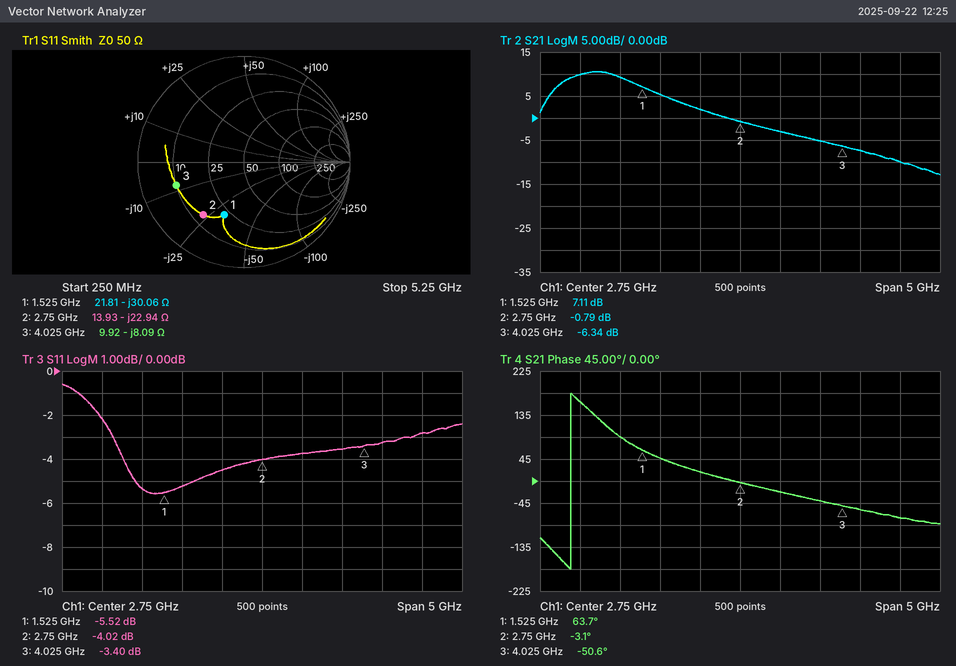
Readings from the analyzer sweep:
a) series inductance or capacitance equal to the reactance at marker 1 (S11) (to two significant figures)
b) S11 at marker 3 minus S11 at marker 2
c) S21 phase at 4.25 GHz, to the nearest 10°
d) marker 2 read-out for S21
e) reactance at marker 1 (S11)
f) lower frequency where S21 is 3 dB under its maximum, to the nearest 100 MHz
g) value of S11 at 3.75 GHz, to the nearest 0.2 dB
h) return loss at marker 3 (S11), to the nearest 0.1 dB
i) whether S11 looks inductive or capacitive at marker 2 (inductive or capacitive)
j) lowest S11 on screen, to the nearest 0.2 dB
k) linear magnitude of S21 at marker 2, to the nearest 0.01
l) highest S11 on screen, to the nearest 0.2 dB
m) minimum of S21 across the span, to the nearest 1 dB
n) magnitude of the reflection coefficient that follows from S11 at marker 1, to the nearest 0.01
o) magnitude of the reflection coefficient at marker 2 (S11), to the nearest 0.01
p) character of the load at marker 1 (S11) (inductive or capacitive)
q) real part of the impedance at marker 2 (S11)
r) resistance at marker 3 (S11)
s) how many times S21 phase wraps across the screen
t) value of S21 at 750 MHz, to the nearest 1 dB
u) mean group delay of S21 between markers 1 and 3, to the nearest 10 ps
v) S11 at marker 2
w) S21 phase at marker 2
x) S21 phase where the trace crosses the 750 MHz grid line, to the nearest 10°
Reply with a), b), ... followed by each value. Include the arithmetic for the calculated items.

a) C = 1/(2π × 1.525 GHz × 30.06 Ω) ≈ 3.5 pF
b) -3.4 − (-4.02) = 0.62 dB
c) -60°
d) -0.79 dB
e) -30.06 Ω
f) 500 MHz
g) -3.6 dB
h) 3.4 dB
i) capacitive
j) -5.6 dB
k) 10^(-0.79/20) ≈ 0.91
l) -0.6 dB
m) -13 dB
n) 10^(-5.52/20) ≈ 0.53
o) 0.63
p) capacitive
q) 13.93 Ω
r) 9.92 Ω
s) 1
t) 10 dB
u) −(-50.6° − (63.7°))/(360° × 2.5 GHz) ≈ 127 ps, so 130 ps to the nearest 10 ps
v) -4.02 dB
w) -3.1°
x) 160°
